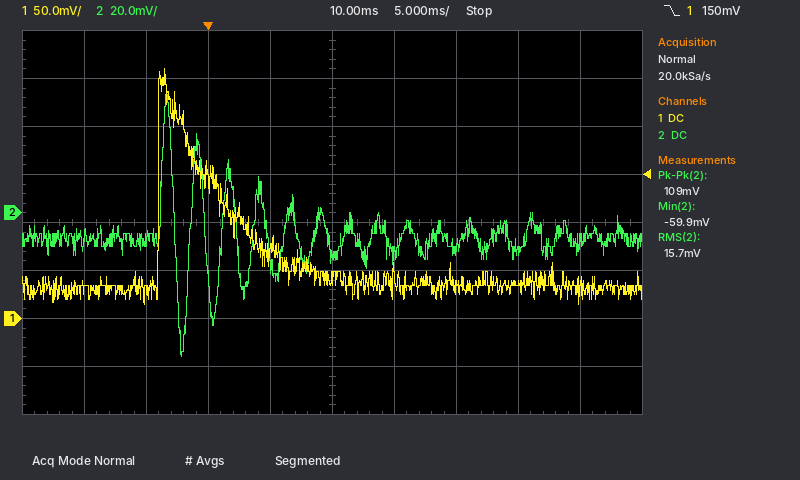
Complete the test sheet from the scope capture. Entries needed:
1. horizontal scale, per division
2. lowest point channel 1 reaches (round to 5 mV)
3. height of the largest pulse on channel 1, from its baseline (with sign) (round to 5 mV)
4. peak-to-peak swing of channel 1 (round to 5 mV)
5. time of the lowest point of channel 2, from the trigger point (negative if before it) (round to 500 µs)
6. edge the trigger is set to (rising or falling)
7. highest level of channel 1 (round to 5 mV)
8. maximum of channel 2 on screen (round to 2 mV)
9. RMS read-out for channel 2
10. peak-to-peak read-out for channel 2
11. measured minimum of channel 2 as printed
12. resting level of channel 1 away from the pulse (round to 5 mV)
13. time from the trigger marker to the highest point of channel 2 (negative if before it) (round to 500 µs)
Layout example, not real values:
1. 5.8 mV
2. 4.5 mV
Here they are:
1. 5 ms
2. 15 mV
3. +225 mV
4. 245 mV
5. -2.0 ms
6. falling
7. 260 mV
8. 50 mV
9. 15.7 mV
10. 109 mV
11. -59.9 mV
12. 35 mV
13. -3.5 ms
